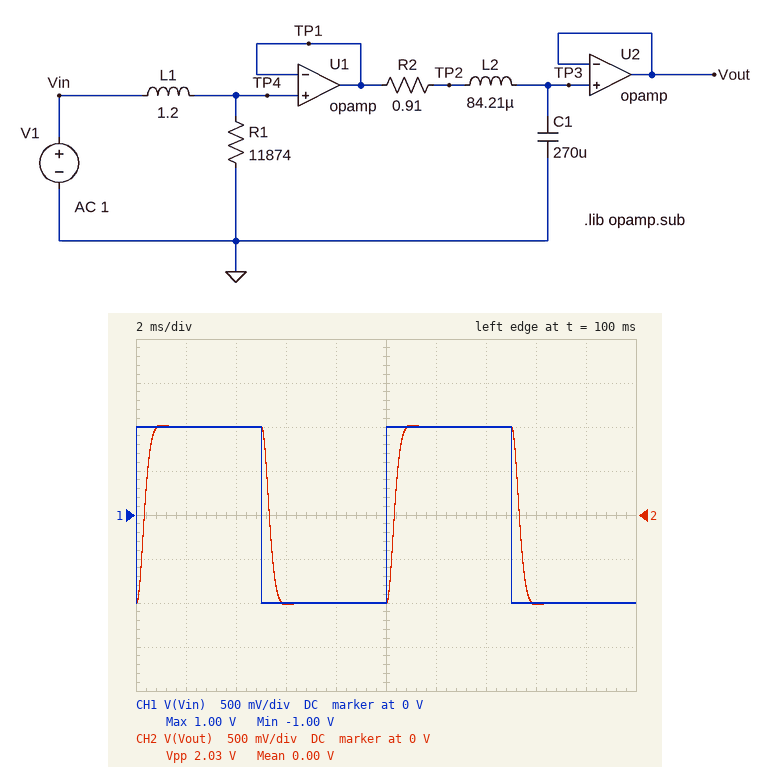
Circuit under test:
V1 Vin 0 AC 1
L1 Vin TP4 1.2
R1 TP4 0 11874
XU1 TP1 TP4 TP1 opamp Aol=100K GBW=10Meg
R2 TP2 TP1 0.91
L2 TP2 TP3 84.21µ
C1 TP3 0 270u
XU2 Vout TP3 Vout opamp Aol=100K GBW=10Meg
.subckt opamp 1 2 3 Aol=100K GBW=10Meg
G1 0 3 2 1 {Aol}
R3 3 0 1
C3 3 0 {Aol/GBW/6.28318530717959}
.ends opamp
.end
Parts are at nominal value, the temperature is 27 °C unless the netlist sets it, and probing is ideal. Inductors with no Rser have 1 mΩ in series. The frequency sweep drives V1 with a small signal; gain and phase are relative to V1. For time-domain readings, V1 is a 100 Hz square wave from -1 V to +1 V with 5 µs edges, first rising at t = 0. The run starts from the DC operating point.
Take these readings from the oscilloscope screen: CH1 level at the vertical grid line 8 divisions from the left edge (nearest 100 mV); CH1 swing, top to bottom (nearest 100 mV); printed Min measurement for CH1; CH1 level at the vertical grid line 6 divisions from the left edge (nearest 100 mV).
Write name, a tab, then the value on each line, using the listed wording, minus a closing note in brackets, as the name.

CH1 level at the vertical grid line 8 divisions from the left edge	-1.0 V
CH1 swing, top to bottom	2.0 V
printed Min measurement for CH1	-1.00 V
CH1 level at the vertical grid line 6 divisions from the left edge	1.0 V
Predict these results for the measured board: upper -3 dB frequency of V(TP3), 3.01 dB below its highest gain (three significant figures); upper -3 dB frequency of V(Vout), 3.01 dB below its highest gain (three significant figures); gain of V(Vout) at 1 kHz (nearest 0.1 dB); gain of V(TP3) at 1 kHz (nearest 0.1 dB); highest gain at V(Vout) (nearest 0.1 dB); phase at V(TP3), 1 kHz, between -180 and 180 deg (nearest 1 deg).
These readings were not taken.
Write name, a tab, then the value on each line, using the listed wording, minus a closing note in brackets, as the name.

upper -3 dB frequency of V(TP3), 3.01 dB below its highest gain	763 Hz
upper -3 dB frequency of V(Vout), 3.01 dB below its highest gain	763 Hz
gain of V(Vout) at 1 kHz	-5.3 dB
gain of V(TP3) at 1 kHz	-5.3 dB
highest gain at V(Vout)	0 dB
phase at V(TP3), 1 kHz, between -180 and 180 deg	-119 deg
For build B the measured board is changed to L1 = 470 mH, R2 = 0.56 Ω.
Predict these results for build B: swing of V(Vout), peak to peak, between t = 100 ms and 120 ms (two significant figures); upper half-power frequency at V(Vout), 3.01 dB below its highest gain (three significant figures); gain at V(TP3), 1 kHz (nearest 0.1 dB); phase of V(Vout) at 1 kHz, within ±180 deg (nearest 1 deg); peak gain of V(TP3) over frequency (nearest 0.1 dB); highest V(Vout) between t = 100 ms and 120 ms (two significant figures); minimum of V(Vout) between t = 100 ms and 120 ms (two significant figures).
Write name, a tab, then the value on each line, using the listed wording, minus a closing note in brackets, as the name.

swing of V(Vout), peak to peak, between t = 100 ms and 120 ms	2.6 V
upper half-power frequency at V(Vout), 3.01 dB below its highest gain	1.21 kHz
gain at V(TP3), 1 kHz	0.1 dB
phase of V(Vout) at 1 kHz, within ±180 deg	-98 deg
peak gain of V(TP3) over frequency	1.1 dB
highest V(Vout) between t = 100 ms and 120 ms	1.3 V
minimum of V(Vout) between t = 100 ms and 120 ms	-1.3 V
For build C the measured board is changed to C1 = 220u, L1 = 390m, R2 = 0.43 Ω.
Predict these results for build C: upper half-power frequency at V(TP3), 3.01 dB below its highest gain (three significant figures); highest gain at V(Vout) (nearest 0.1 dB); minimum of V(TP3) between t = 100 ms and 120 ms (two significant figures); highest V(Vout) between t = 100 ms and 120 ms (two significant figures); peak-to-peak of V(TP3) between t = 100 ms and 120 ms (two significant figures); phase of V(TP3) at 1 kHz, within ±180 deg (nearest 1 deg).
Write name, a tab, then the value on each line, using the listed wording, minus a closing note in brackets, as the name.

upper half-power frequency at V(TP3), 3.01 dB below its highest gain	1.38 kHz
highest gain at V(Vout)	3.5 dB
minimum of V(TP3) between t = 100 ms and 120 ms	-1.6 V
highest V(Vout) between t = 100 ms and 120 ms	1.6 V
peak-to-peak of V(TP3) between t = 100 ms and 120 ms	3.2 V
phase of V(TP3) at 1 kHz, within ±180 deg	-77 deg
